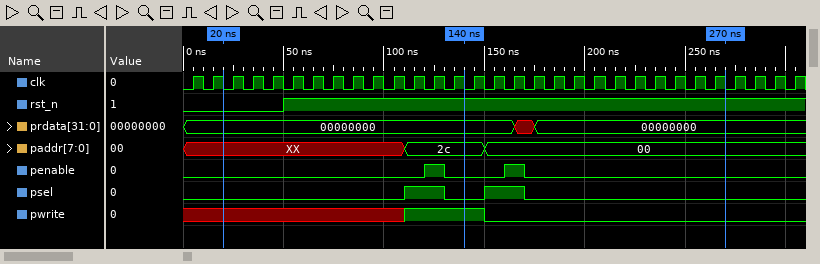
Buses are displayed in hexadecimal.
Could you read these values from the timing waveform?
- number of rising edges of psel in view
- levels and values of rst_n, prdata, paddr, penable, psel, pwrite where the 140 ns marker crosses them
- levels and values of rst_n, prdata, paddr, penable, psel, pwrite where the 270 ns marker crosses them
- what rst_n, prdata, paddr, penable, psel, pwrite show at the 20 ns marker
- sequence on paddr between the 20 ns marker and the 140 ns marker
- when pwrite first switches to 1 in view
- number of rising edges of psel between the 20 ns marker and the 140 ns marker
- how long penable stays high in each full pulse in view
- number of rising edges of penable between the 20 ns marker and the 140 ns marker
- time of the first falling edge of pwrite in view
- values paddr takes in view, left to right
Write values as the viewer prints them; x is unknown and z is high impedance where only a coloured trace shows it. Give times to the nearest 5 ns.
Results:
2
rst_n=1, prdata=00000000, paddr=2c, penable=0, psel=0, pwrite=1
rst_n=1, prdata=00000000, paddr=00, penable=0, psel=0, pwrite=0
rst_n=0, prdata=00000000, paddr=XX, penable=0, psel=0, pwrite=x
XX, 2c
110 ns
1
10 ns, 10 ns
1
150 ns
XX, 2c, 00
